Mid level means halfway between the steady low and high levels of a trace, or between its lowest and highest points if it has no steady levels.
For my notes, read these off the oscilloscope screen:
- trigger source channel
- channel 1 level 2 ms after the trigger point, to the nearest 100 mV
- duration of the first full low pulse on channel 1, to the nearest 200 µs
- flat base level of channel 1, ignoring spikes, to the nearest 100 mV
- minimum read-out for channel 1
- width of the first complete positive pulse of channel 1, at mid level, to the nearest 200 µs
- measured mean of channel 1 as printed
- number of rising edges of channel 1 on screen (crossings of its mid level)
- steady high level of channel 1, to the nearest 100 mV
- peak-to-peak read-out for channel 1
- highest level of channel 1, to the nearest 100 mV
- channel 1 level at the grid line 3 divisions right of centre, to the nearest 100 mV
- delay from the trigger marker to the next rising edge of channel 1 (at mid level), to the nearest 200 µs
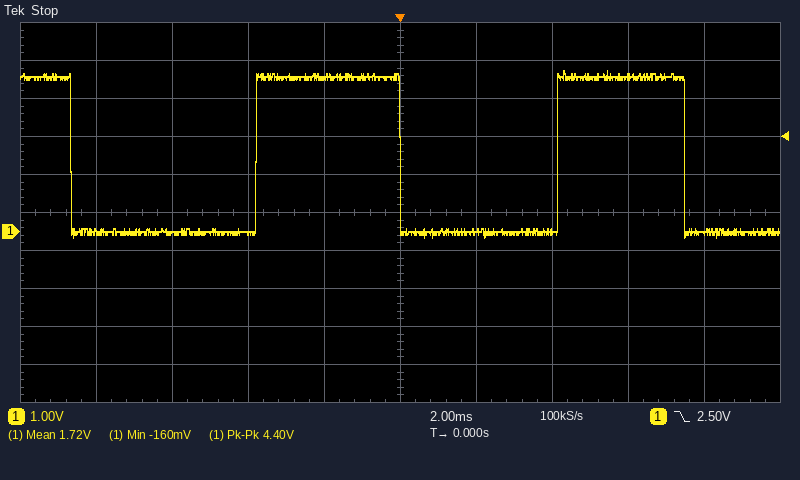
channel 1
0.0 V
4.8 ms
0.0 V
-160 mV
3.8 ms
1.72 V
2
4.1 V
4.40 V
4.2 V
4.1 V
4.2 ms
